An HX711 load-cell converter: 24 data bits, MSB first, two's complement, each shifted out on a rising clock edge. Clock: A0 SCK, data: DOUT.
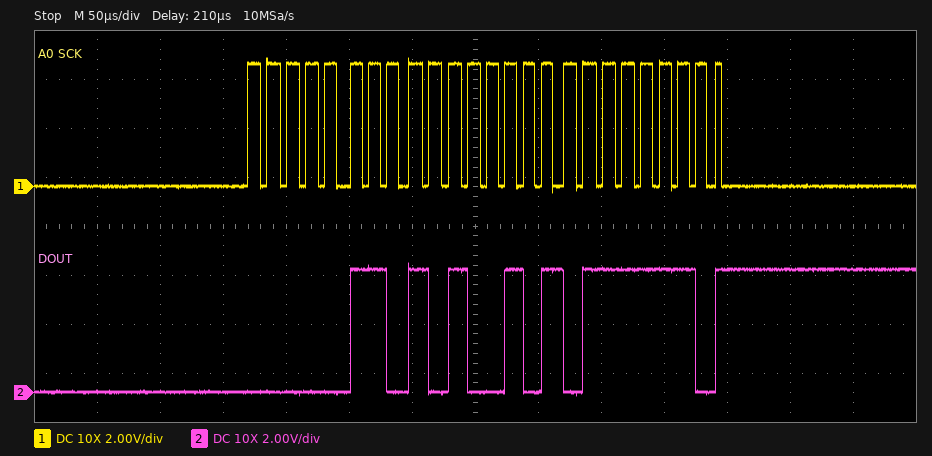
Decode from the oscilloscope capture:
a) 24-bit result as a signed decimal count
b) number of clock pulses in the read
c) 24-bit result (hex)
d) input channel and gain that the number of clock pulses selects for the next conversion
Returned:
435582
25
0x06A57E
channel A, gain 128
